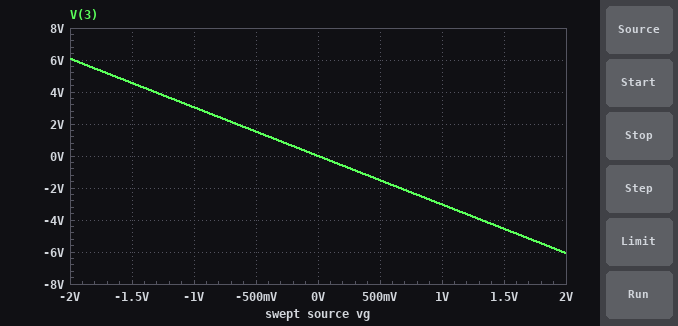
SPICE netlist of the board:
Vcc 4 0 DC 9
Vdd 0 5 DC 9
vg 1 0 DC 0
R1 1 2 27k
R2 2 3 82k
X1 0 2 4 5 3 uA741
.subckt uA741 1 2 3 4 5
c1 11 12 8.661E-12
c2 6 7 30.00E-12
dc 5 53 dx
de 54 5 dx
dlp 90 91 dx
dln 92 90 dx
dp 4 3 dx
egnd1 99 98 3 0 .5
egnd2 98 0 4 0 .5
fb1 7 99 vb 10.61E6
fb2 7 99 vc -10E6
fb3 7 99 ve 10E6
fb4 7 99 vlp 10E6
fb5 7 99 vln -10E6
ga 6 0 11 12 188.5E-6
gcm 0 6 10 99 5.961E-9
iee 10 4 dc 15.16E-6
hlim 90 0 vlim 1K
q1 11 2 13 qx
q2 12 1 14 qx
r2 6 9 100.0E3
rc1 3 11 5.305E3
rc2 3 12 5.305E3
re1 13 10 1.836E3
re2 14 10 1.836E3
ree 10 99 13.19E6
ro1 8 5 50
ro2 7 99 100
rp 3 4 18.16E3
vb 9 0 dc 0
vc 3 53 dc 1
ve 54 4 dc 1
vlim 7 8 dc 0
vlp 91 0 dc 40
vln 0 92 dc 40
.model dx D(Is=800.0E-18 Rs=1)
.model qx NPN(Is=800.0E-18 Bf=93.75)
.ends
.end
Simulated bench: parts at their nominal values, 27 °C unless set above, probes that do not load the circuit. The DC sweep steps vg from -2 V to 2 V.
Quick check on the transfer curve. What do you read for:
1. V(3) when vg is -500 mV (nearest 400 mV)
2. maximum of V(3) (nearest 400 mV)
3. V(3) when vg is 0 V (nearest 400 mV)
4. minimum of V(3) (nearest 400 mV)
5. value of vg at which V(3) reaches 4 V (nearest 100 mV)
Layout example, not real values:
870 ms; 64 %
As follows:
1.6 V; 6.0 V; 0 V; -6.0 V; -1.3 V
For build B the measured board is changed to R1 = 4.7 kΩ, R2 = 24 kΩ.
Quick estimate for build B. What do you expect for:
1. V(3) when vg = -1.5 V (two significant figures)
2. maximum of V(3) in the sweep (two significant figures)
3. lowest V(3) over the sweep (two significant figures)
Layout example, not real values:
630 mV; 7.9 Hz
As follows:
7.7 V; 8.6 V; -8.6 V
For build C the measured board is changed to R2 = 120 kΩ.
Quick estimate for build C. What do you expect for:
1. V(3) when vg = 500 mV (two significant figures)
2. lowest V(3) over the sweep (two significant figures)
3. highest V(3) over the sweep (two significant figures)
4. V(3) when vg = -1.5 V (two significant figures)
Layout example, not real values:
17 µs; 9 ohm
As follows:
-2.2 V; -8.6 V; 8.6 V; 6.7 V
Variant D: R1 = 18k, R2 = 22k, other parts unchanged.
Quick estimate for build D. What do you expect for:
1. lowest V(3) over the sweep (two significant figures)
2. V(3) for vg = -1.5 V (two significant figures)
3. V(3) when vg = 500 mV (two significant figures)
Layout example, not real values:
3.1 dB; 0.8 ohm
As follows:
-2.4 V; 1.8 V; -610 mV
